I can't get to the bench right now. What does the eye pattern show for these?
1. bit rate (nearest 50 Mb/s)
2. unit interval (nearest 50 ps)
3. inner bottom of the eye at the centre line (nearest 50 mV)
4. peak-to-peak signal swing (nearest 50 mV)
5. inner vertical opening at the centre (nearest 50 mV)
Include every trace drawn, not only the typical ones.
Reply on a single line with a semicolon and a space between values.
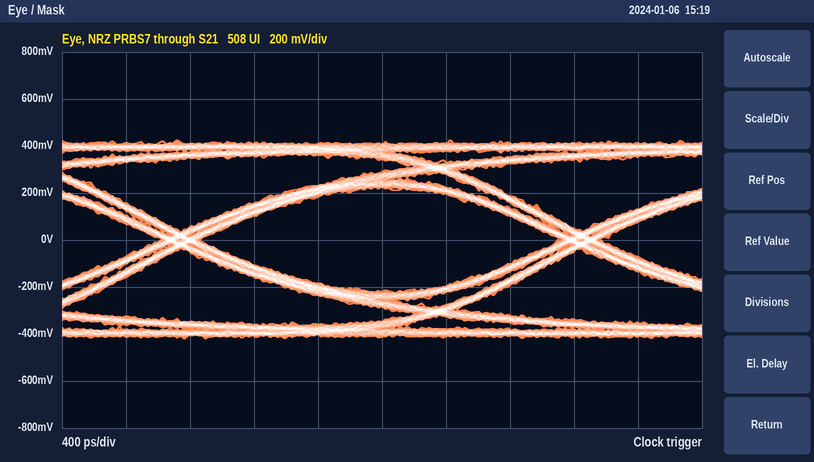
400 Mb/s; 2.50 ns; -200 mV; 850 mV; 450 mV
